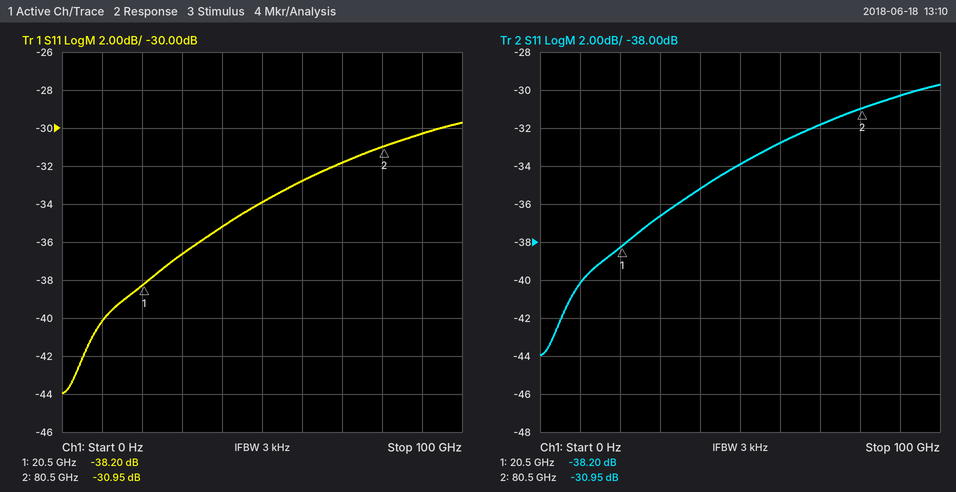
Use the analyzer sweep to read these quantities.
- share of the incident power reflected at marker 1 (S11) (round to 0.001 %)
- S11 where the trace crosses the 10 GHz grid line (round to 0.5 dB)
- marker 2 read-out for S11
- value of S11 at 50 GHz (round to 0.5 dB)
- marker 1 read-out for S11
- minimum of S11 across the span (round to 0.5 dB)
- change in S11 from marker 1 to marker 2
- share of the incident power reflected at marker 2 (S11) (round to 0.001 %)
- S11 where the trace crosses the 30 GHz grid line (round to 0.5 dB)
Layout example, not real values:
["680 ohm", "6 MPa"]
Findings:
["0.015 %", "-40.0 dB", "-30.95 dB", "-34.0 dB", "-38.20 dB", "-44.0 dB", "7.25 dB", "0.080 %", "-36.5 dB"]
